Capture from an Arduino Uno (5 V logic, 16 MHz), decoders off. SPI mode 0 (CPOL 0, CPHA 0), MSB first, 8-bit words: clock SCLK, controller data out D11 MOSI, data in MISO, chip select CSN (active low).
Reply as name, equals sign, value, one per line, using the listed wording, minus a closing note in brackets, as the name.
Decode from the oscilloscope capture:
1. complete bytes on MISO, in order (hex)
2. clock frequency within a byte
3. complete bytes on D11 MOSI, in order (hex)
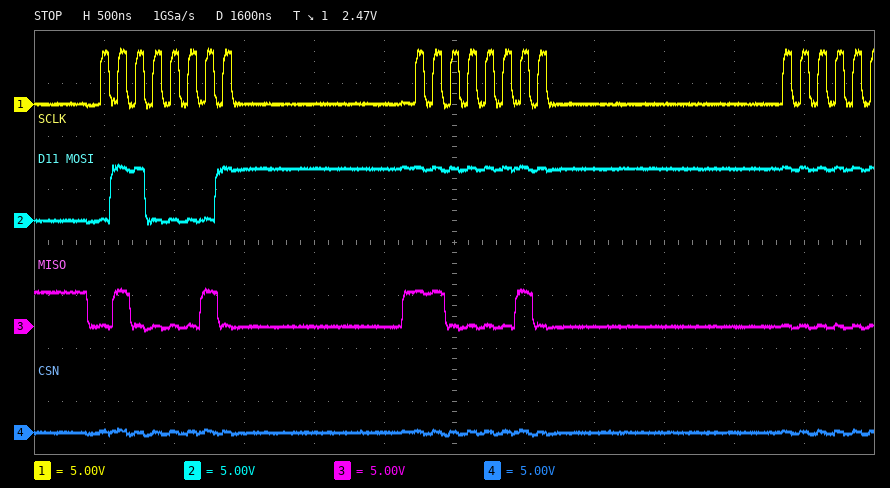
complete bytes on MISO, in order = 42 C2
clock frequency within a byte = 8 MHz
complete bytes on D11 MOSI, in order = 61 FF
